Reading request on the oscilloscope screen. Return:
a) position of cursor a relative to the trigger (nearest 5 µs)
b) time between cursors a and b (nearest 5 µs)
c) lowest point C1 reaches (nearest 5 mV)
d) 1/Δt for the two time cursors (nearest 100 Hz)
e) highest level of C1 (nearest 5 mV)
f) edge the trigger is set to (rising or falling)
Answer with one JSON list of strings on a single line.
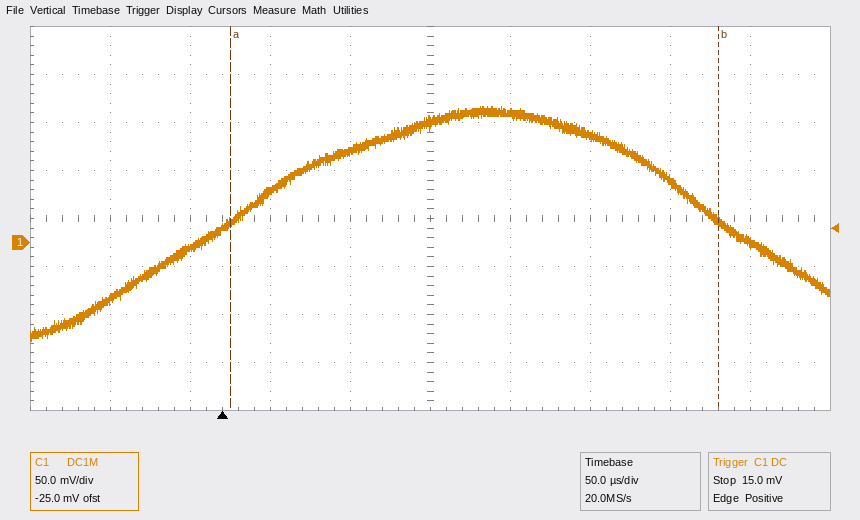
["+5 µs", "305 µs", "-100 mV", "3.3 kHz", "140 mV", "rising"]
